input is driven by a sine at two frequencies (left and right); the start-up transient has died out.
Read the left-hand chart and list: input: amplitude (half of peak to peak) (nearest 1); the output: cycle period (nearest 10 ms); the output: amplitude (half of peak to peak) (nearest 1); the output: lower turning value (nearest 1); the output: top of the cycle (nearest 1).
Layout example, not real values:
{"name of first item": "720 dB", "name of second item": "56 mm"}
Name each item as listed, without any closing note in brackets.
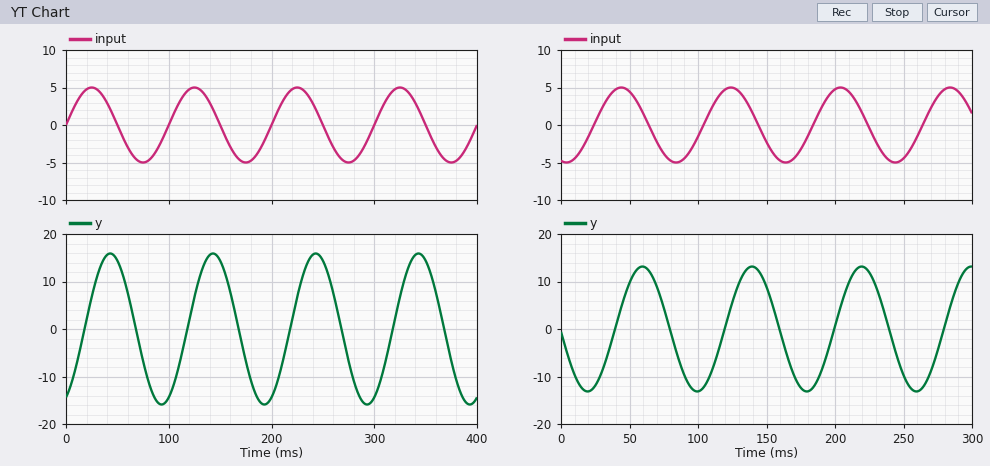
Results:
{"input: amplitude (half of peak to peak)": "5", "the output: cycle period": "100 ms", "the output: amplitude (half of peak to peak)": "16", "the output: lower turning value": "-16", "the output: top of the cycle": "16"}
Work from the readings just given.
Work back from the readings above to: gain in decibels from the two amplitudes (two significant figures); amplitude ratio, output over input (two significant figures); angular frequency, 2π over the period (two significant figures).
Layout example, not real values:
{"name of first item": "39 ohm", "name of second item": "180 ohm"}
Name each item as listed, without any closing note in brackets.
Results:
{"gain in decibels from the two amplitudes": "10 dB", "amplitude ratio, output over input": "3.2", "angular frequency, 2π over the period": "0.063 rad/ms"}
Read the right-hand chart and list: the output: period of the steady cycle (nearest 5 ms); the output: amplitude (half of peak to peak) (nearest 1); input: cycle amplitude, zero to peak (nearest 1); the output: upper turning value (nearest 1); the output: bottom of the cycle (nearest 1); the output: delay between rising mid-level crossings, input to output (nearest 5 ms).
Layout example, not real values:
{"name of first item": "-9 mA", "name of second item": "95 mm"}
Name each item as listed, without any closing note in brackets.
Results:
{"the output: period of the steady cycle": "80 ms", "the output: amplitude (half of peak to peak)": "13", "input: cycle amplitude, zero to peak": "5", "the output: upper turning value": "13", "the output: bottom of the cycle": "-13", "the output: delay between rising mid-level crossings, input to output": "15 ms"}
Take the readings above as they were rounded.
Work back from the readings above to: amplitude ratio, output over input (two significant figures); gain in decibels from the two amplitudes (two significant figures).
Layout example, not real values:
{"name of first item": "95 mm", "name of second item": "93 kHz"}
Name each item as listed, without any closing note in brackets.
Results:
{"amplitude ratio, output over input": "2.6", "gain in decibels from the two amplitudes": "8.3 dB"}
